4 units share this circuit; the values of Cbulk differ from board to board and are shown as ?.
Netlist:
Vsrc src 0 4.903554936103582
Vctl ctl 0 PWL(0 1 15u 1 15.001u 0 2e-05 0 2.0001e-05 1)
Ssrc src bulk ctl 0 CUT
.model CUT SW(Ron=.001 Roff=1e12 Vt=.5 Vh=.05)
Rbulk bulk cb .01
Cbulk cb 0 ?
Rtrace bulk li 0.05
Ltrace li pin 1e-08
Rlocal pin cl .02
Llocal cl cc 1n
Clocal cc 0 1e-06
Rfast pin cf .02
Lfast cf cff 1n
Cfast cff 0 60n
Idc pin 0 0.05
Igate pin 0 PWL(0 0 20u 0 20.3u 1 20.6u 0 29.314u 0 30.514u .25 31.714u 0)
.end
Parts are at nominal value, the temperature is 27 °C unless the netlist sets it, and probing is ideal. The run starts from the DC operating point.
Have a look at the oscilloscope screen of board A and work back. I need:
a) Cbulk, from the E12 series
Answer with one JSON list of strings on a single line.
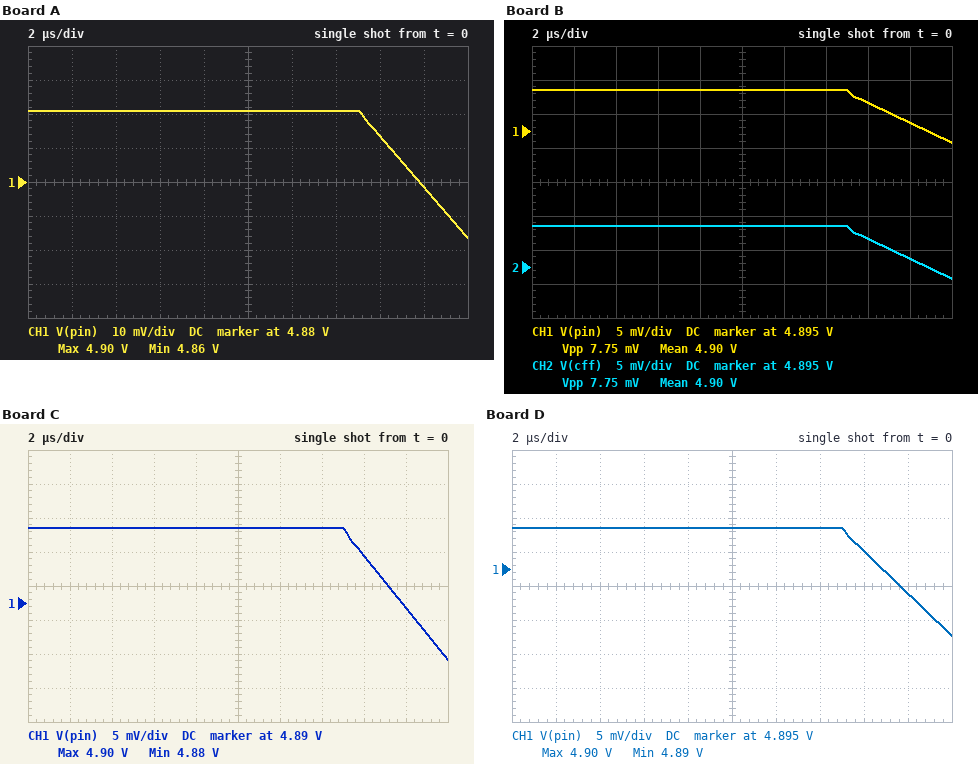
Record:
["5.6 µF"]
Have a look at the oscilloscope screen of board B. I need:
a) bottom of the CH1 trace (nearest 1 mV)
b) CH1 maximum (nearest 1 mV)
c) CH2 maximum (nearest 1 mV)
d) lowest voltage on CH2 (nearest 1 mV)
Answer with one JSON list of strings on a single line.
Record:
["4.893 V", "4.901 V", "4.901 V", "4.893 V"]
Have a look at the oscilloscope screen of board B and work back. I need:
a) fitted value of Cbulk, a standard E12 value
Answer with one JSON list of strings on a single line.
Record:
["33 µF"]
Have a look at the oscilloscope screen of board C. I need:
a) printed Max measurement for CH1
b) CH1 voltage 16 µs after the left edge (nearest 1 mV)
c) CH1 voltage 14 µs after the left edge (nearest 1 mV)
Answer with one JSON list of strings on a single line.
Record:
["4.90 V", "4.897 V", "4.901 V"]
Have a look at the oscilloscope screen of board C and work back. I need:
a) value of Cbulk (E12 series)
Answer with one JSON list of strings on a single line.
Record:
["12 µF"]
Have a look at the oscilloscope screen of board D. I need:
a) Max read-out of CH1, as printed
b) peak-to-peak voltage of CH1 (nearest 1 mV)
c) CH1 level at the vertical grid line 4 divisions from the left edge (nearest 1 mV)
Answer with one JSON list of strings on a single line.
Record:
["4.90 V", "16 mV", "4.901 V"]
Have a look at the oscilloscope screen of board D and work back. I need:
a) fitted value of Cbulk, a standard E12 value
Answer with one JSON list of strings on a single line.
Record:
["15 µF"]
